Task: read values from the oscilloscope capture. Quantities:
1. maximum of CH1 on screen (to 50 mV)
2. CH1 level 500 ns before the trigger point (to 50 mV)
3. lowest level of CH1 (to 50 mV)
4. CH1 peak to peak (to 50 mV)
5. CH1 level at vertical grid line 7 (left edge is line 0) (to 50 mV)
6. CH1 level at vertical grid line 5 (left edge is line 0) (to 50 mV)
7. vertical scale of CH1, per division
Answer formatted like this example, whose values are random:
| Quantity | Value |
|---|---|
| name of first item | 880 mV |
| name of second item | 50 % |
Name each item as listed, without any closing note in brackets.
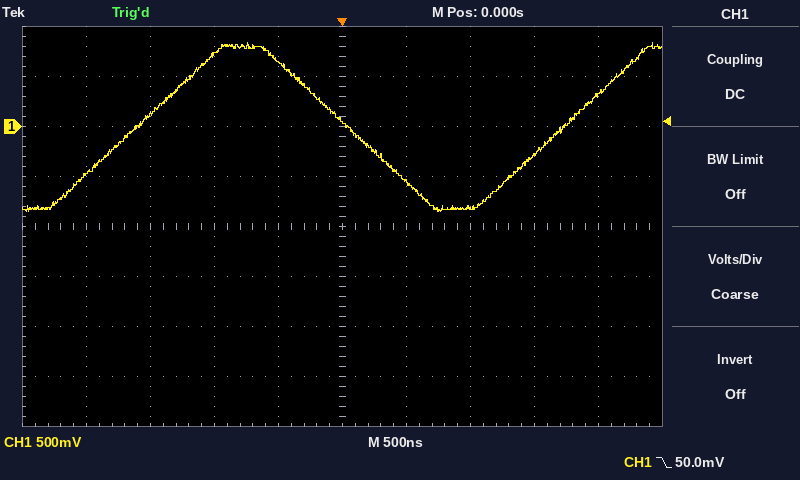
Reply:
| Quantity | Value |
|---|---|
| maximum of CH1 on screen | 850 mV |
| CH1 level 500 ns before the trigger point | 650 mV |
| lowest level of CH1 | -850 mV |
| CH1 peak to peak | 1.70 V |
| CH1 level at vertical grid line 7 (left edge is line 0) | -800 mV |
| CH1 level at vertical grid line 5 (left edge is line 0) | 50 mV |
| vertical scale of CH1, per division | 500 mV |
